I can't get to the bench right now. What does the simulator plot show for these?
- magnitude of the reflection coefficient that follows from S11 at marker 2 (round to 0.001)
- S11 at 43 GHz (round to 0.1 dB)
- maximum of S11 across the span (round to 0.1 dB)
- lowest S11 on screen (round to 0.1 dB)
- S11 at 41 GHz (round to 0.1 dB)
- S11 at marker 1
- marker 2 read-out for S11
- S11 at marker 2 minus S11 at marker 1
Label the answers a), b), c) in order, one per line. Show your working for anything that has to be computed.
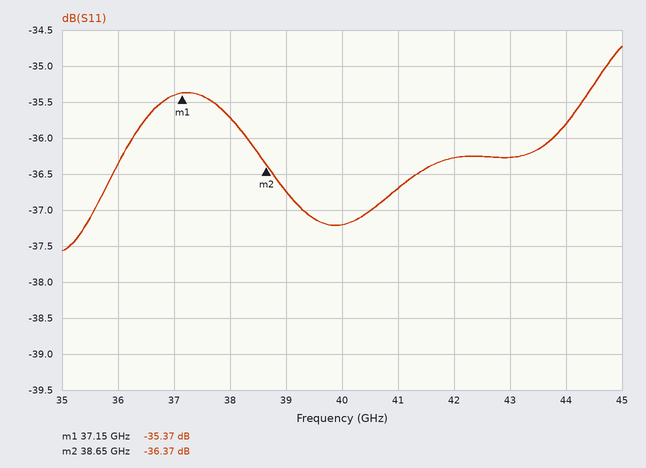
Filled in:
a) 10^(-36.37/20) ≈ 0.015
b) -36.3 dB
c) -34.7 dB
d) -37.6 dB
e) -36.7 dB
f) -35.37 dB
g) -36.37 dB
h) -36.37 − (-35.37) = -1.00 dB
